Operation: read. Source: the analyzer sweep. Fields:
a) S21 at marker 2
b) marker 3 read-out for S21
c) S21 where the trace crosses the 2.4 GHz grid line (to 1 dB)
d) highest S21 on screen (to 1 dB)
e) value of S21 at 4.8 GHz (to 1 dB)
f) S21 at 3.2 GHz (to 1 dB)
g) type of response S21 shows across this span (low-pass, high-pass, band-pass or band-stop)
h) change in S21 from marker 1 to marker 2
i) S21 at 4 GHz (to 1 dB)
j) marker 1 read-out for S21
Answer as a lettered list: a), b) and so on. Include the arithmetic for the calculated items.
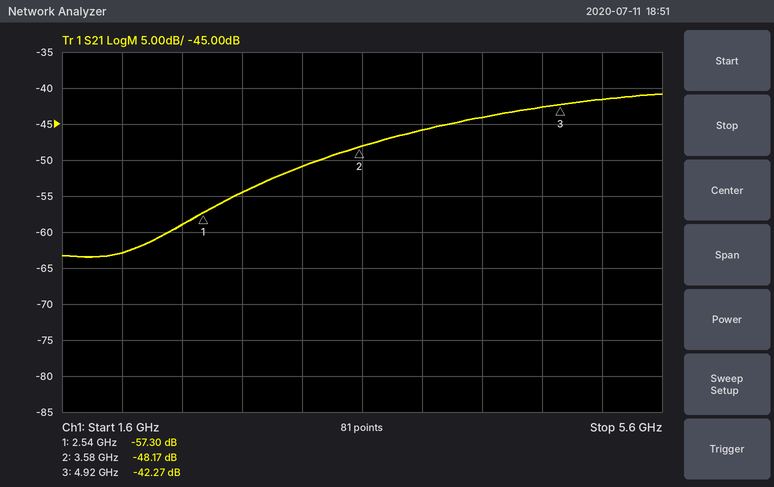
a) -48.17 dB
b) -42.27 dB
c) -59 dB
d) -41 dB
e) -43 dB
f) -51 dB
g) high-pass
h) -48.17 − (-57.3) = 9.13 dB
i) -46 dB
j) -57.30 dB
